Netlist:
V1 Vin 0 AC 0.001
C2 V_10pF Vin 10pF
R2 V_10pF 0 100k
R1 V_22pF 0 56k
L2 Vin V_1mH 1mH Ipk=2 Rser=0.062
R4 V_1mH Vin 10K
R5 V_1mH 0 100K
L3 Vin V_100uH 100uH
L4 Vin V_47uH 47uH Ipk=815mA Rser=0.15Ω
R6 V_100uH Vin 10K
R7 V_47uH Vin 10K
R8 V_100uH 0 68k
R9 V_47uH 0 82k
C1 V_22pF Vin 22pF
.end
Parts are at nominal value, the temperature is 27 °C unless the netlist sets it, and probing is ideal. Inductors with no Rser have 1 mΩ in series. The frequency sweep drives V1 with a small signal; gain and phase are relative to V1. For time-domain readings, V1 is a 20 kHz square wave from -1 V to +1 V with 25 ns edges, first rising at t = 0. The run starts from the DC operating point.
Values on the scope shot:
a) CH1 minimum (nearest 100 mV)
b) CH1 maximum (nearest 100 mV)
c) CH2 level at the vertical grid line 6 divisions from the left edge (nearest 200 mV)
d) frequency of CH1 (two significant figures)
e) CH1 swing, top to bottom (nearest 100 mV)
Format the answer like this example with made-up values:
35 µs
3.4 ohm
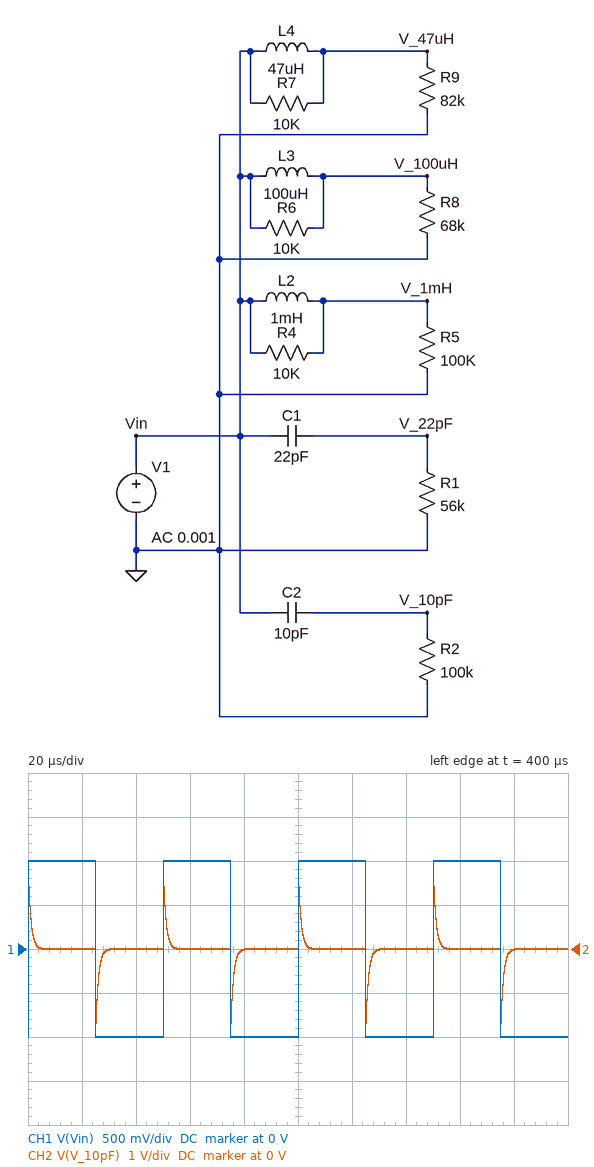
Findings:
-1.0 V
1.0 V
0 V
20 kHz
2.0 V
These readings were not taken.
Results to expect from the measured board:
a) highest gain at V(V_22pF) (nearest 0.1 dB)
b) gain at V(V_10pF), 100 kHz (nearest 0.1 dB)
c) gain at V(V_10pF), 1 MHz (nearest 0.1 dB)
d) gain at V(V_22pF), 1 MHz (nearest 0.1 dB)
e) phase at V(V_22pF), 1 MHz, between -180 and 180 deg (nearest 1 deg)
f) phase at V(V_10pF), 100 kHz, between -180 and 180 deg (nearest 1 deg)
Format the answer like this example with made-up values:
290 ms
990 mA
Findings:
0 dB
-5.5 dB
-0.1 dB
-0.1 dB
7 deg
58 deg
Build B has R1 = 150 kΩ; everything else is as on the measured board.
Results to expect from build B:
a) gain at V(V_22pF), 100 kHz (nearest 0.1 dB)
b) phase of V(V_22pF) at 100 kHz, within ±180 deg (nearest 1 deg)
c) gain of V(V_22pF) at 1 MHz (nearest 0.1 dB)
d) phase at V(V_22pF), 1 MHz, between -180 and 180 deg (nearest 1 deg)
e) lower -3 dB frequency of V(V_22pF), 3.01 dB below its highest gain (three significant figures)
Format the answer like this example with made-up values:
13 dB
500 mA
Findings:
-0.9 dB
26 deg
0 dB
3 deg
48.2 kHz
